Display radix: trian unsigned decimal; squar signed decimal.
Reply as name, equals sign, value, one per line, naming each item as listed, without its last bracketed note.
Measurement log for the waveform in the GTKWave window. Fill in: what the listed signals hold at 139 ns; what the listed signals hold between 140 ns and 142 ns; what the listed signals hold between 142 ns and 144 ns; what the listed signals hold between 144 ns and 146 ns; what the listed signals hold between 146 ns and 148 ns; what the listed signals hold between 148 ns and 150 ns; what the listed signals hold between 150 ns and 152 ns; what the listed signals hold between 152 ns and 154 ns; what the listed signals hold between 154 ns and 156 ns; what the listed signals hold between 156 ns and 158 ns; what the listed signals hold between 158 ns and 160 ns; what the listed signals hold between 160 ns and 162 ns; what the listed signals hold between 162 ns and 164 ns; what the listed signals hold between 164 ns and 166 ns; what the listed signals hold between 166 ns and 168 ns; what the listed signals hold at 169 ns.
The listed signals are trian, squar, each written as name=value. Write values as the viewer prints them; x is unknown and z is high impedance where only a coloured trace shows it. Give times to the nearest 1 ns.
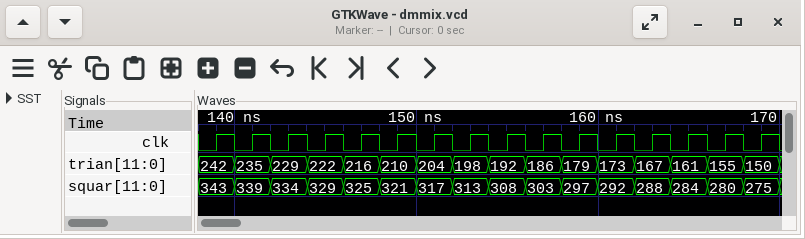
what the listed signals hold at 139 ns = trian=242, squar=343
what the listed signals hold between 140 ns and 142 ns = trian=235, squar=339
what the listed signals hold between 142 ns and 144 ns = trian=229, squar=334
what the listed signals hold between 144 ns and 146 ns = trian=222, squar=329
what the listed signals hold between 146 ns and 148 ns = trian=216, squar=325
what the listed signals hold between 148 ns and 150 ns = trian=210, squar=321
what the listed signals hold between 150 ns and 152 ns = trian=204, squar=317
what the listed signals hold between 152 ns and 154 ns = trian=198, squar=313
what the listed signals hold between 154 ns and 156 ns = trian=192, squar=308
what the listed signals hold between 156 ns and 158 ns = trian=186, squar=303
what the listed signals hold between 158 ns and 160 ns = trian=179, squar=297
what the listed signals hold between 160 ns and 162 ns = trian=173, squar=292
what the listed signals hold between 162 ns and 164 ns = trian=167, squar=288
what the listed signals hold between 164 ns and 166 ns = trian=161, squar=284
what the listed signals hold between 166 ns and 168 ns = trian=155, squar=280
what the listed signals hold at 169 ns = trian=150, squar=275
